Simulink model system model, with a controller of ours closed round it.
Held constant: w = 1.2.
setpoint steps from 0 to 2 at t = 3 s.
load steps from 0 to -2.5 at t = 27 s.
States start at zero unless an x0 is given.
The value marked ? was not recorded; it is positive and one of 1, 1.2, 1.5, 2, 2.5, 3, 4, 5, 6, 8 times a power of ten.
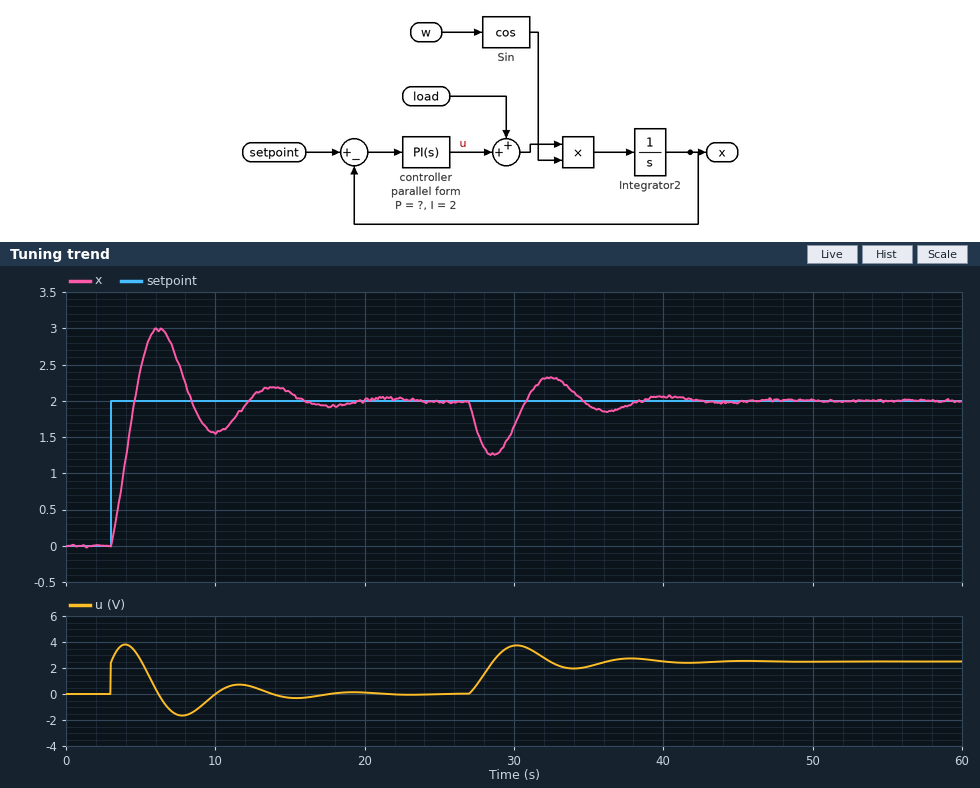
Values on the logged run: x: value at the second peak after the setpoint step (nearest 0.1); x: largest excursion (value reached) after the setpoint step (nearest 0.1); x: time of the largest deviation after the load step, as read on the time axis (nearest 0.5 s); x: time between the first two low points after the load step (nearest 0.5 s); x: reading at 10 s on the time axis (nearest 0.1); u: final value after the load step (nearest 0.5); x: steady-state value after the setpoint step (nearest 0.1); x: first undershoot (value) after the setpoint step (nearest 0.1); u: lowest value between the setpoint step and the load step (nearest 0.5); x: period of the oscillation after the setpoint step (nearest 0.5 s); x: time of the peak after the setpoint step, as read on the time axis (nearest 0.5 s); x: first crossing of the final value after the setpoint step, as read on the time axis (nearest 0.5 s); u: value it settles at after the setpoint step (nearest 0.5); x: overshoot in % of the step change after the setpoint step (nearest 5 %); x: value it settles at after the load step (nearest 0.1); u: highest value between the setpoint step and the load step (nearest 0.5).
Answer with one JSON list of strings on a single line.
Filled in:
["2.2", "3.0", "28.5 s", "7.5 s", "1.6", "2.5", "2.0", "1.6", "-1.5", "7.5 s", "6.0 s", "4.5 s", "0.0", "50 %", "2.0", "4.0"]
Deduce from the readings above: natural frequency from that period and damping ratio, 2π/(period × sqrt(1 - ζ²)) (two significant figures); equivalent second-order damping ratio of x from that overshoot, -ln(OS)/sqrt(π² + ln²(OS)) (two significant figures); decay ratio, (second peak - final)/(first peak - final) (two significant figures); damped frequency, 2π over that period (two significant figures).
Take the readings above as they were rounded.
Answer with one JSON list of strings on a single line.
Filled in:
["0.86 rad/s", "0.22", "0.20", "0.84 rad/s"]
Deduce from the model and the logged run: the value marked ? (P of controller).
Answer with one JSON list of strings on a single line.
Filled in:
["1.2"]
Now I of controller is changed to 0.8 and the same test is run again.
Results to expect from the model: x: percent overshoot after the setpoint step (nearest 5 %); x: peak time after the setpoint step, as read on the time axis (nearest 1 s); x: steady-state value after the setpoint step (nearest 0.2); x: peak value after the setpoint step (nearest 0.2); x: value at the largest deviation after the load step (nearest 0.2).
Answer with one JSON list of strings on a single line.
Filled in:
["35 %", "8 s", "2.0", "2.8", "1.0"]
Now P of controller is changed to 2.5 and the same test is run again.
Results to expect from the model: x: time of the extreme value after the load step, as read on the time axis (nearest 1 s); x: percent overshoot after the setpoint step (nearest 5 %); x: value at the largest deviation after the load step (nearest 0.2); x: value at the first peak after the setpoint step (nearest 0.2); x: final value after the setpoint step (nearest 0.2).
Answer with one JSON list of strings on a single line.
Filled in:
["28 s", "30 %", "1.4", "2.6", "2.0"]
